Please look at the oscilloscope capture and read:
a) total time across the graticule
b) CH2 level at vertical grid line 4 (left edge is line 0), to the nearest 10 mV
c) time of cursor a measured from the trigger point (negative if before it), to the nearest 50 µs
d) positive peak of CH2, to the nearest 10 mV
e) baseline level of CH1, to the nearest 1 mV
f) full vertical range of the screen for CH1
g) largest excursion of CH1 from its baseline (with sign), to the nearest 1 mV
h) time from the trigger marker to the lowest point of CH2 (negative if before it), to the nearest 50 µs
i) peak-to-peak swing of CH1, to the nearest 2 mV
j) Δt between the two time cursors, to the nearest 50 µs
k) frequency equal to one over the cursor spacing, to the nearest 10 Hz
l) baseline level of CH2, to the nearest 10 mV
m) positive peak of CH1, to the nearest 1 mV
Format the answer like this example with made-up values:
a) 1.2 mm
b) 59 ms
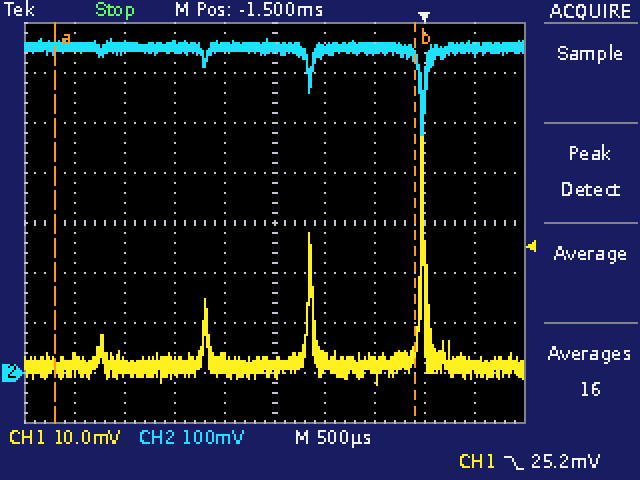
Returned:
a) 5 ms
b) 650 mV
c) -3.70 ms
d) 670 mV
e) 1 mV
f) 80 mV
g) +46 mV
h) 0 µs
i) 50 mV
j) 3.60 ms
k) 280 Hz
l) 650 mV
m) 47 mV
